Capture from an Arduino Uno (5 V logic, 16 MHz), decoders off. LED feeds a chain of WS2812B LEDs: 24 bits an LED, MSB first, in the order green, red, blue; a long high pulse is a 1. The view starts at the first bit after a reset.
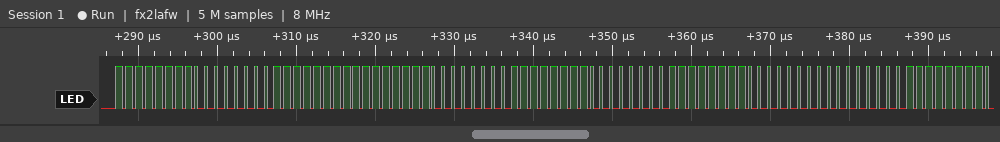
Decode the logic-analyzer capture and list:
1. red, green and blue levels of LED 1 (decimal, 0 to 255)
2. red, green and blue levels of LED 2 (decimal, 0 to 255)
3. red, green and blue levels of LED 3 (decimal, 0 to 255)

0, 255, 255
0, 255, 255
255, 0, 0
